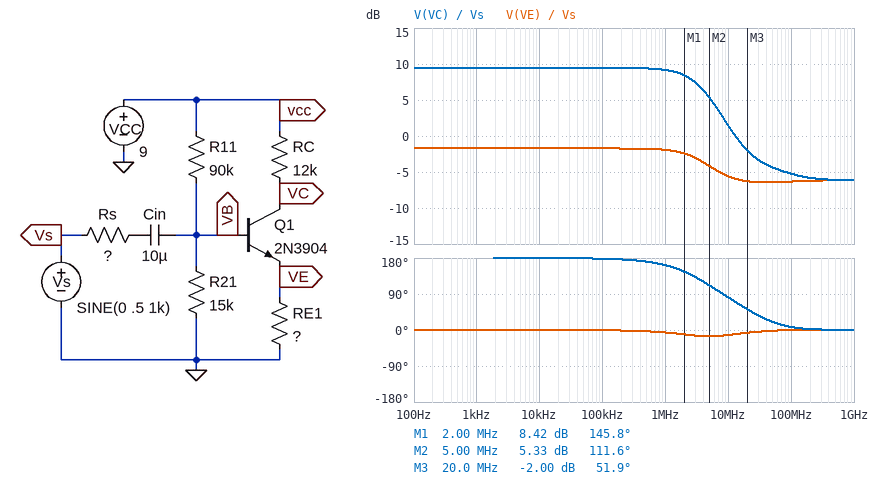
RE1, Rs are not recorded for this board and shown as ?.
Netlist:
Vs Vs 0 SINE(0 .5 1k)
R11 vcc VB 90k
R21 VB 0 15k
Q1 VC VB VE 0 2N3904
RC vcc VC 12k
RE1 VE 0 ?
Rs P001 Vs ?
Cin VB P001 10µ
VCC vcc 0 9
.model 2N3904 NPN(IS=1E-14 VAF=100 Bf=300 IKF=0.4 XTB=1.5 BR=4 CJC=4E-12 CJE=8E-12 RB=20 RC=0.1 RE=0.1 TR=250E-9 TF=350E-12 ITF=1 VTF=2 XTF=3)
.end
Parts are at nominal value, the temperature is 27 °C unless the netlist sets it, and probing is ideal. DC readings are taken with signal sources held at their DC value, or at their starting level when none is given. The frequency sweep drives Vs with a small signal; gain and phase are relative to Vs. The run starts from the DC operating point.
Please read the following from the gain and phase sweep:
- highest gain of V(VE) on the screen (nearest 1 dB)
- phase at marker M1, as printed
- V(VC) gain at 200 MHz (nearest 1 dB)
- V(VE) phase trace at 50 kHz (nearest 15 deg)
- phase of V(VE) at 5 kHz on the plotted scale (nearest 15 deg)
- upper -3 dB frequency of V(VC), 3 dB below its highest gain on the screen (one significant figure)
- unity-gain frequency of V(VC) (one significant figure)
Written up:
-2 dB
145.8 deg
-6 dB
0 deg
0 deg
4 MHz
10 MHz
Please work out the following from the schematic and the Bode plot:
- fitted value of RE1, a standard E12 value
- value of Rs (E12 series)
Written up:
3.3 kΩ
2.2 kΩ
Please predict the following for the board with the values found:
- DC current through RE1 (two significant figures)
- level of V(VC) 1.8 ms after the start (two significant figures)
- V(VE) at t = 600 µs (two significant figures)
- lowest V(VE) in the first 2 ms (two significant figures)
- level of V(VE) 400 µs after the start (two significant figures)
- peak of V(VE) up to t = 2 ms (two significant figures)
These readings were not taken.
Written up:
200 µA
8.0 V
430 mV
260 mV
910 mV
1.1 V
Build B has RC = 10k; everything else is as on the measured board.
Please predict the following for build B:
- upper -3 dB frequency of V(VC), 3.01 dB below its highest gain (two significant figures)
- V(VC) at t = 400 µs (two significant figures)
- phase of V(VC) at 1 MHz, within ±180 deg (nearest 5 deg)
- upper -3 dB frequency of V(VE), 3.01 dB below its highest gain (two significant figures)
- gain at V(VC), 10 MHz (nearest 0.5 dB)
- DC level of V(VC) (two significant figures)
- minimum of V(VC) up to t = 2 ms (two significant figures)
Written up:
4.8 MHz
6.3 V
165 deg
7.3 MHz
1.0 dB
7.0 V
5.7 V
